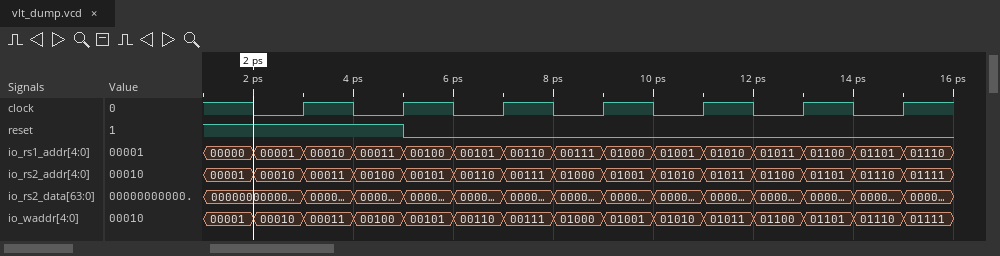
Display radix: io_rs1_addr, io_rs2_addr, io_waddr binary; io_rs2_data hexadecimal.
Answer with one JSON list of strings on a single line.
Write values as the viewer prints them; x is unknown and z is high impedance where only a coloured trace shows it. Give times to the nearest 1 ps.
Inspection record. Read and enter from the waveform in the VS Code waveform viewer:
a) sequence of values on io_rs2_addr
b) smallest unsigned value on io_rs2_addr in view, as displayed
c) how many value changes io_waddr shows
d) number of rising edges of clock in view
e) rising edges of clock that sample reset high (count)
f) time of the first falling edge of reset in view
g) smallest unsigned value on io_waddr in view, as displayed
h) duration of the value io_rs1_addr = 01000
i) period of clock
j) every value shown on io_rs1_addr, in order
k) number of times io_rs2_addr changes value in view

["00001, 00010, 00011, 00100, 00101, 00110, 00111, 01000, 01001, 01010, 01011, 01100, 01101, 01110, 01111", "00001", "14", "7", "2", "5 ps", "00001", "1 ps", "2 ps", "00000, 00001, 00010, 00011, 00100, 00101, 00110, 00111, 01000, 01001, 01010, 01011, 01100, 01101, 01110", "14"]
